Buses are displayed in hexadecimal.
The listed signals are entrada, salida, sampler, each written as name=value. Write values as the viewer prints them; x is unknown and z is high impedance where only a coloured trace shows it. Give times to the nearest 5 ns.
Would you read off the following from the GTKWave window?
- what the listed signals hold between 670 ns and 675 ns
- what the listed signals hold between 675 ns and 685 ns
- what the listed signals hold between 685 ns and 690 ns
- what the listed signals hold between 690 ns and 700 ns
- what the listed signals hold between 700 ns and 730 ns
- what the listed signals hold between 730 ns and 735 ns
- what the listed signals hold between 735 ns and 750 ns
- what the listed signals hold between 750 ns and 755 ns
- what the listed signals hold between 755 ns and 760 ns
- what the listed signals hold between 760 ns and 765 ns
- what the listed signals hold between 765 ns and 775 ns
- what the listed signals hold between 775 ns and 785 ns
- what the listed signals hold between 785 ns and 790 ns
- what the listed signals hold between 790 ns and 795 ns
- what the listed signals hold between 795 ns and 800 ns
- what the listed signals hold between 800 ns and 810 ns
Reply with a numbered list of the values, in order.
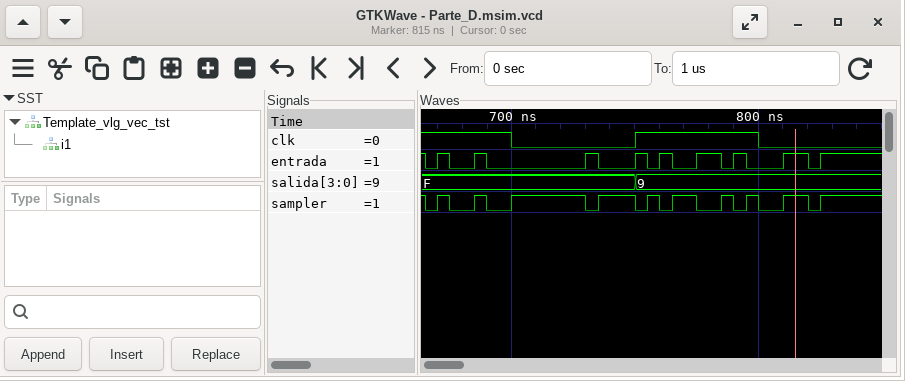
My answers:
1. entrada=1, salida=F, sampler=1
2. entrada=0, salida=F, sampler=0
3. entrada=1, salida=F, sampler=1
4. entrada=0, salida=F, sampler=0
5. entrada=0, salida=F, sampler=1
6. entrada=1, salida=F, sampler=0
7. entrada=0, salida=F, sampler=1
8. entrada=1, salida=9, sampler=0
9. entrada=0, salida=9, sampler=1
10. entrada=1, salida=9, sampler=0
11. entrada=0, salida=9, sampler=1
12. entrada=1, salida=9, sampler=0
13. entrada=0, salida=9, sampler=1
14. entrada=1, salida=9, sampler=0
15. entrada=0, salida=9, sampler=1
16. entrada=0, salida=9, sampler=0
